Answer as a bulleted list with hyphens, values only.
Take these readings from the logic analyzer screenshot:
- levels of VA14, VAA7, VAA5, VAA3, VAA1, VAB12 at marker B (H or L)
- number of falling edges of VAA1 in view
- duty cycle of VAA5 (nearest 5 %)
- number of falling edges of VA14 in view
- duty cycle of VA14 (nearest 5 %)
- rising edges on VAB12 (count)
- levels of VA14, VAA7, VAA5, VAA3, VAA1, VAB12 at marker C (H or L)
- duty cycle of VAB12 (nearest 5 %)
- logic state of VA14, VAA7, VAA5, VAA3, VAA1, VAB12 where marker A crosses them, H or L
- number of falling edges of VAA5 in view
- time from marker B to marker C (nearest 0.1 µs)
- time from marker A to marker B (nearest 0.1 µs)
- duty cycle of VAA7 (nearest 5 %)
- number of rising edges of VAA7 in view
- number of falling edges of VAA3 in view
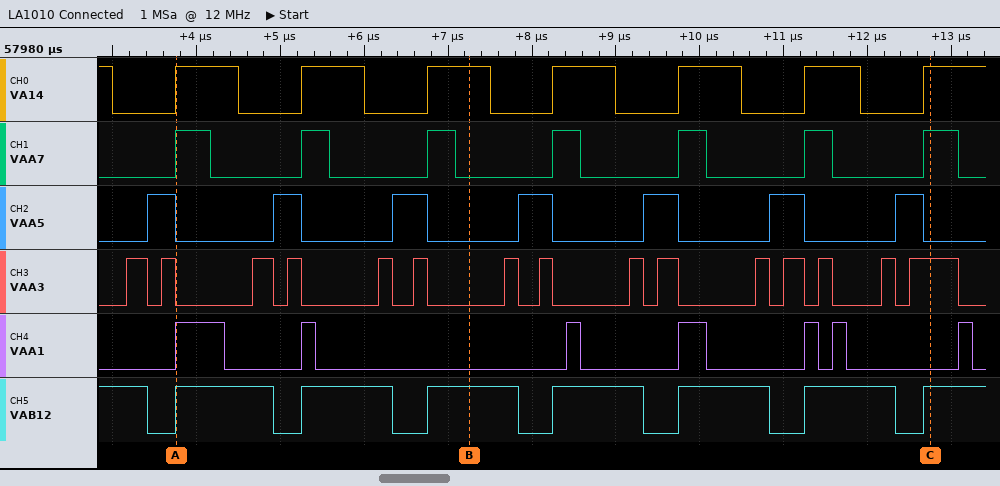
- VA14=H, VAA7=L, VAA5=L, VAA3=L, VAA1=L, VAB12=H
- 7
- 25 %
- 7
- 50 %
- 7
- VA14=H, VAA7=H, VAA5=L, VAA3=H, VAA1=L, VAB12=H
- 75 %
- VA14=H, VAA7=H, VAA5=L, VAA3=L, VAA1=H, VAB12=H
- 7
- 5.5 µs
- 3.5 µs
- 25 %
- 7
- 15
